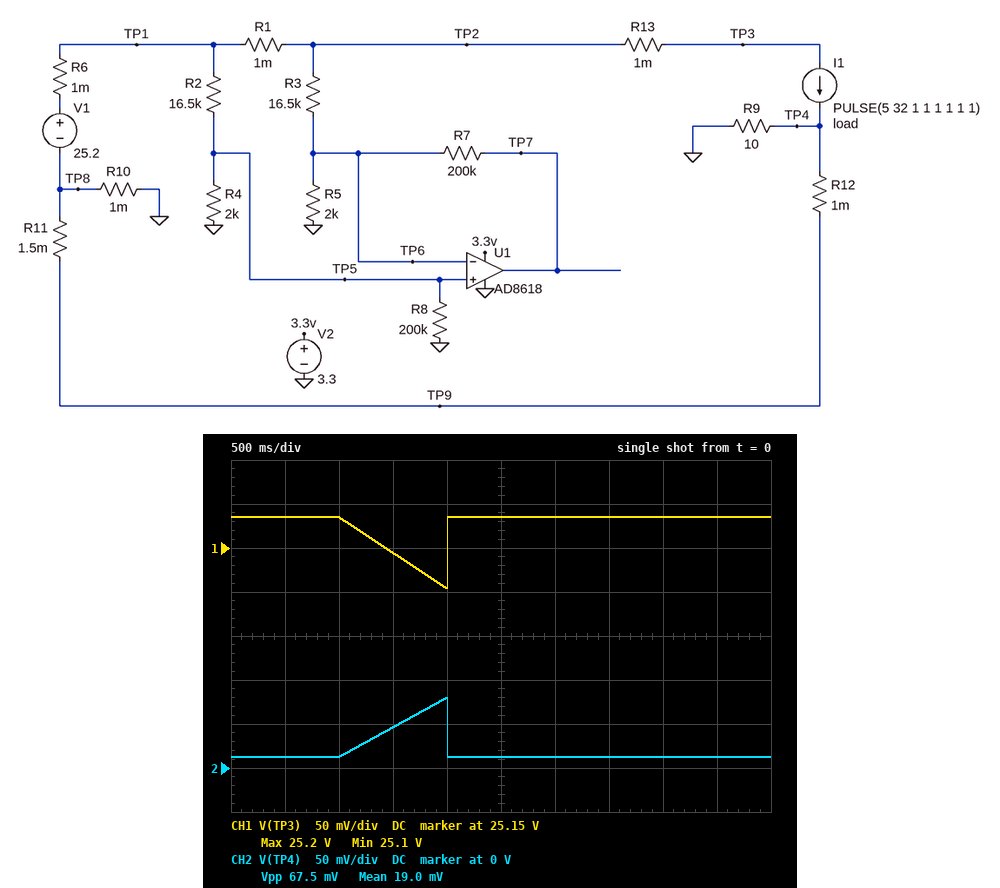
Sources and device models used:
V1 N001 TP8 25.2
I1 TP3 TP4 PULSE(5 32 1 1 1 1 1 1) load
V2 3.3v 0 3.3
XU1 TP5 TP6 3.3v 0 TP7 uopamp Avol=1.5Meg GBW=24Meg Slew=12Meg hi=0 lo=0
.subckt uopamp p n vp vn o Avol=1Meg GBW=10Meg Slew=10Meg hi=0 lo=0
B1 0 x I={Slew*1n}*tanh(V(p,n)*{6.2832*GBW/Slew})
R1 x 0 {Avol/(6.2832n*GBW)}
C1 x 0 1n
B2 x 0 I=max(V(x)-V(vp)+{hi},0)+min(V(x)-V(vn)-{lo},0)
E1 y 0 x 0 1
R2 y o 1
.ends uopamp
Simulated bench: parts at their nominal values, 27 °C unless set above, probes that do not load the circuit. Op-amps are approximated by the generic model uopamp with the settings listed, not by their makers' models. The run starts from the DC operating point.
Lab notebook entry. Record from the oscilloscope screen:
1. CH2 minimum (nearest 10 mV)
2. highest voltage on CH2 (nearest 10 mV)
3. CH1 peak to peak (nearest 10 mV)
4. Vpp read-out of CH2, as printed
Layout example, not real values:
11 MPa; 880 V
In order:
10 mV; 80 mV; 80 mV; 67.5 mV
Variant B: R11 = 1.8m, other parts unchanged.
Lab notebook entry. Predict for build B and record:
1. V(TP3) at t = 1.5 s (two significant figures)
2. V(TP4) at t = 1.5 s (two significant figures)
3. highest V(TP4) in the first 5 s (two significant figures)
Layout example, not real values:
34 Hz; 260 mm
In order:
25 V; 52 mV; 90 mV
